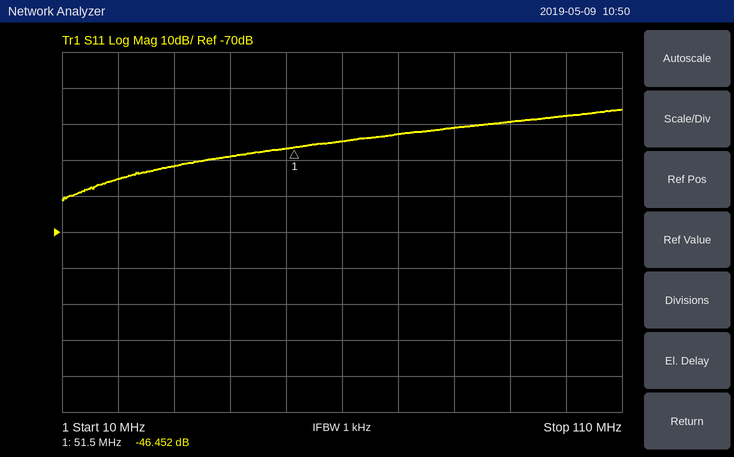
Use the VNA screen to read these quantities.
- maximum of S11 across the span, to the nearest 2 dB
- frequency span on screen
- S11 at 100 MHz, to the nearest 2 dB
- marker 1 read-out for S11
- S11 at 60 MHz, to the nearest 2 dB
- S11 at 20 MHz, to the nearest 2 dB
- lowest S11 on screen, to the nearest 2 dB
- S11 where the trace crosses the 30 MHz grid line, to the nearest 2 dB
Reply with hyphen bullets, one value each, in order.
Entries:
- -36 dB
- 100 MHz
- -38 dB
- -46.452 dB
- -44 dB
- -56 dB
- -62 dB
- -52 dB
